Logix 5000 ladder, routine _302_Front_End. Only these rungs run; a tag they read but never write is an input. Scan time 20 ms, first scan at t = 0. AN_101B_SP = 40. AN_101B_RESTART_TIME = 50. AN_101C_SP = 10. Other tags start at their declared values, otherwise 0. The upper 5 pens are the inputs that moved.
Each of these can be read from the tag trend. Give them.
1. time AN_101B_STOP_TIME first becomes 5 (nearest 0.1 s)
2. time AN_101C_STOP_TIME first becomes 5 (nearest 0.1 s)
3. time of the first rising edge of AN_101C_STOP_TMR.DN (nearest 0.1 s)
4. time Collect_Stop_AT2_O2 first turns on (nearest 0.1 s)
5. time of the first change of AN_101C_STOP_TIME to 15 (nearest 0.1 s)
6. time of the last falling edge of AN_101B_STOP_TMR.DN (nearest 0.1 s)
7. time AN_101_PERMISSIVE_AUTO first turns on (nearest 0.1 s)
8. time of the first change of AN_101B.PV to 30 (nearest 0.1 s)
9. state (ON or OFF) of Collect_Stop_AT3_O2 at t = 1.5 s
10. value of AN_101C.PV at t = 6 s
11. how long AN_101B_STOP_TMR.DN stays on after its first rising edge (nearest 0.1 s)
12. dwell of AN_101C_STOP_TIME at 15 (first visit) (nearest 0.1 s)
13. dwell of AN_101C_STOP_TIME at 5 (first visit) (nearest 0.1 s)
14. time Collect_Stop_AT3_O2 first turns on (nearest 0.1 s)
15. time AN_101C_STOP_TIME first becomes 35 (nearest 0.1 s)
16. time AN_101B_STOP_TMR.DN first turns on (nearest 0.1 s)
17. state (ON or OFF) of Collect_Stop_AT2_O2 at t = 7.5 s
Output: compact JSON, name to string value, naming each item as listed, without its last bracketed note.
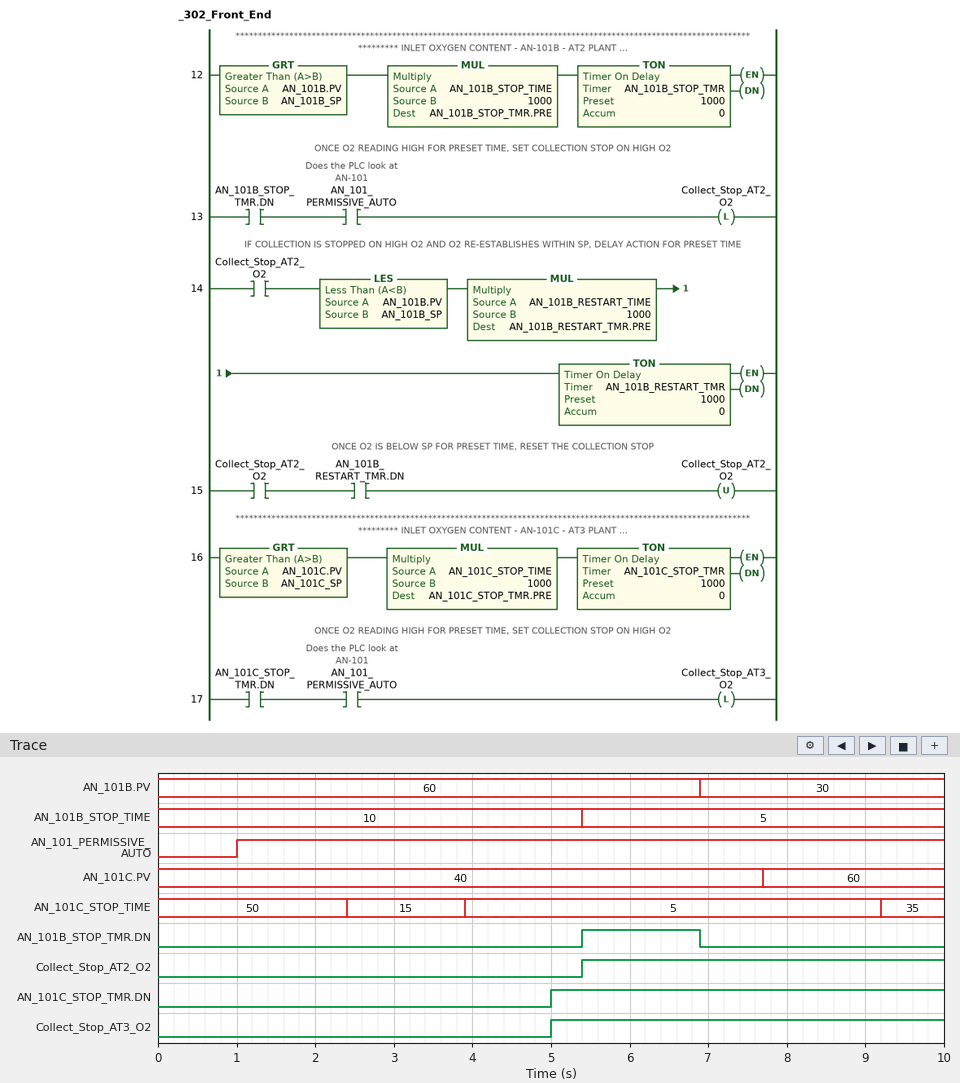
{"time AN_101B_STOP_TIME first becomes 5": "5.4 s", "time AN_101C_STOP_TIME first becomes 5": "3.9 s", "time of the first rising edge of AN_101C_STOP_TMR.DN": "5.0 s", "time Collect_Stop_AT2_O2 first turns on": "5.4 s", "time of the first change of AN_101C_STOP_TIME to 15": "2.4 s", "time of the last falling edge of AN_101B_STOP_TMR.DN": "6.9 s", "time AN_101_PERMISSIVE_AUTO first turns on": "1.0 s", "time of the first change of AN_101B.PV to 30": "6.9 s", "state (ON or OFF) of Collect_Stop_AT3_O2 at t = 1.5 s": "OFF", "value of AN_101C.PV at t = 6 s": "40", "how long AN_101B_STOP_TMR.DN stays on after its first rising edge": "1.5 s", "dwell of AN_101C_STOP_TIME at 15 (first visit)": "1.5 s", "dwell of AN_101C_STOP_TIME at 5 (first visit)": "5.3 s", "time Collect_Stop_AT3_O2 first turns on": "5.0 s", "time AN_101C_STOP_TIME first becomes 35": "9.2 s", "time AN_101B_STOP_TMR.DN first turns on": "5.4 s", "state (ON or OFF) of Collect_Stop_AT2_O2 at t = 7.5 s": "ON"}
